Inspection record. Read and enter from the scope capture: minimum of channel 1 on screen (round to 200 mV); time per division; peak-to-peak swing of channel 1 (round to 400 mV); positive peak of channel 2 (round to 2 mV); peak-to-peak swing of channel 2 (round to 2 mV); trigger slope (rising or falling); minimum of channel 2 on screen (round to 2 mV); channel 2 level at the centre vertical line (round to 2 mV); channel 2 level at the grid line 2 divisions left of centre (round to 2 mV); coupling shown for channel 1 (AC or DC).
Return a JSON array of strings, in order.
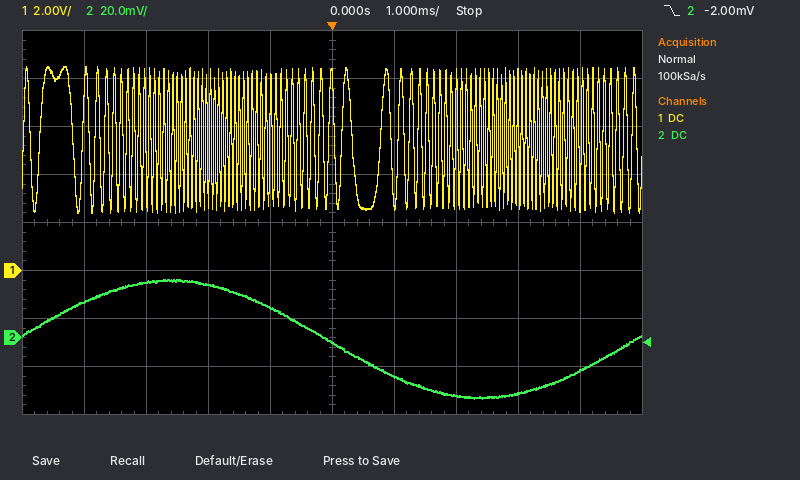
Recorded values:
["2.4 V", "1 ms", "6.0 V", "24 mV", "50 mV", "falling", "-26 mV", "-2 mV", "22 mV", "DC"]
